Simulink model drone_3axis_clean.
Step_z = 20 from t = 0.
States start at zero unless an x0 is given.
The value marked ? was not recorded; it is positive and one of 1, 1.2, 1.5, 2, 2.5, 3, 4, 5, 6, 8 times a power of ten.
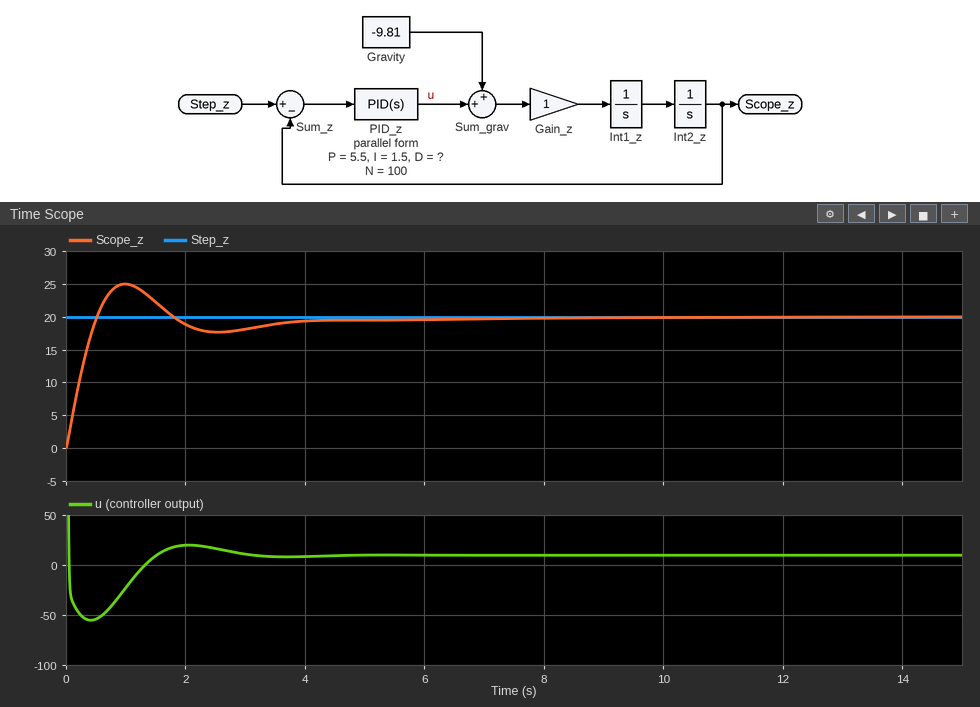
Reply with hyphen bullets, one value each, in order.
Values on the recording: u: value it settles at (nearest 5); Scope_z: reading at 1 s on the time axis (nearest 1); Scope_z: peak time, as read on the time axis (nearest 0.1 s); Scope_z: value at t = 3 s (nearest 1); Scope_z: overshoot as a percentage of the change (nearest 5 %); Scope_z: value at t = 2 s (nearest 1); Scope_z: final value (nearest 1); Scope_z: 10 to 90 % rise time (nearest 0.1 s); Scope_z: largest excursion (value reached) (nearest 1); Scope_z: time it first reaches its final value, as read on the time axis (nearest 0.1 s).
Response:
- 10
- 25
- 1.0 s
- 18
- 25 %
- 19
- 20
- 0.4 s
- 25
- 0.5 s
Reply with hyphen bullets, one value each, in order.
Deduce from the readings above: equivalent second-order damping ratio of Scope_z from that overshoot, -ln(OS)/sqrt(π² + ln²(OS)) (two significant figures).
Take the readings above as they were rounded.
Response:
- 0.40
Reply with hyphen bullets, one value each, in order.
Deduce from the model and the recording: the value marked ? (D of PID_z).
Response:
- 2.5
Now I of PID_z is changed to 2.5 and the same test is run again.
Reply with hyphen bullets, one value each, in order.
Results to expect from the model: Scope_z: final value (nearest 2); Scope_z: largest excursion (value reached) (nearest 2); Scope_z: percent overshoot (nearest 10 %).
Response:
- 20
- 26
- 30 %
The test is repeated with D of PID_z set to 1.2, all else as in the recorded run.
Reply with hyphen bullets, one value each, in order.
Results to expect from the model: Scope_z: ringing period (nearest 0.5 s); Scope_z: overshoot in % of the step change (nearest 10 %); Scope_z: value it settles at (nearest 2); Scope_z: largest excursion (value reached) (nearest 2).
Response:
- 3.0 s
- 50 %
- 20
- 30
